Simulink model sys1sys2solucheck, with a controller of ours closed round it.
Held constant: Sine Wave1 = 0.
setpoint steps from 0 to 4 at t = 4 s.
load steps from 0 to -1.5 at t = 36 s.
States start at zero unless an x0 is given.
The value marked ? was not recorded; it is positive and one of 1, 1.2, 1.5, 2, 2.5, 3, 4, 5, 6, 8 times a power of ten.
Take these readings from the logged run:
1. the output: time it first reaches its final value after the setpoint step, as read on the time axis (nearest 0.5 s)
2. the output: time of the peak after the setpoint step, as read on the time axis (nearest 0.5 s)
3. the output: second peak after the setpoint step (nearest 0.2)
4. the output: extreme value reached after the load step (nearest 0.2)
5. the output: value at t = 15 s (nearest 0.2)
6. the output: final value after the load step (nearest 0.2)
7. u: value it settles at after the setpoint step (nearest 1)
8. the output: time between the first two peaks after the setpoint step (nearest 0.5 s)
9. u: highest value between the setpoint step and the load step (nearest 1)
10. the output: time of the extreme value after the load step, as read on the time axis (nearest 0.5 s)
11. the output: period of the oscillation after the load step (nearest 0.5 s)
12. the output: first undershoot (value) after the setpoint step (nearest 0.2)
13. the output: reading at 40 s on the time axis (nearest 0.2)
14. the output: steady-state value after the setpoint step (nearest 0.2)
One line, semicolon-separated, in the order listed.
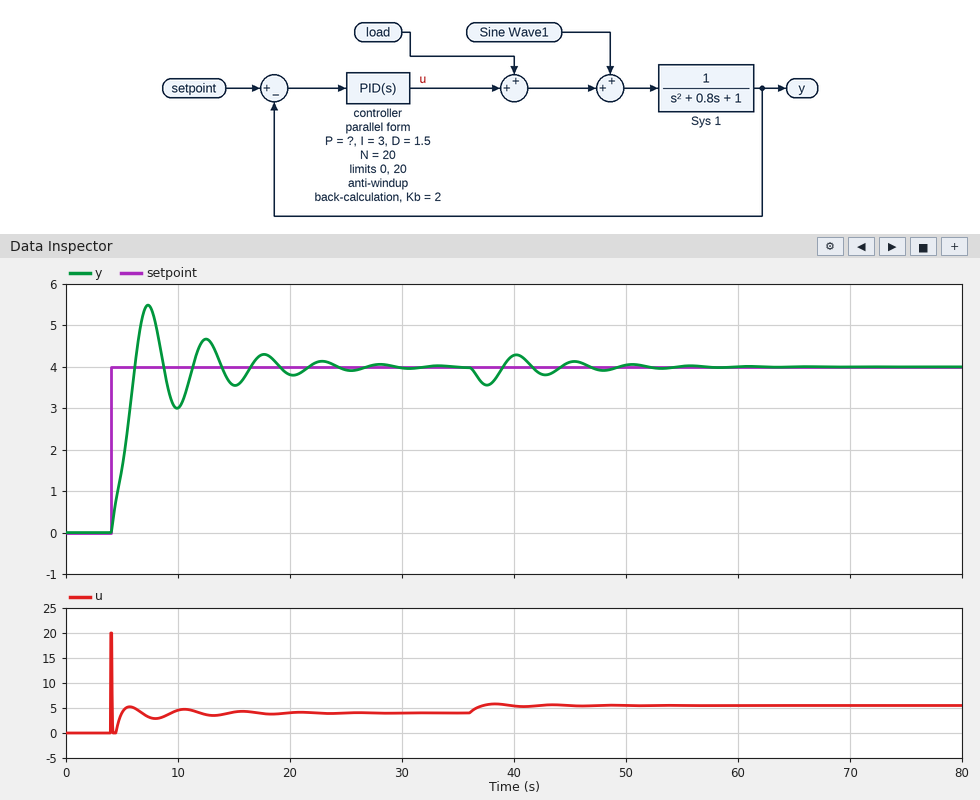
6.0 s; 7.5 s; 4.6; 3.6; 3.6; 4.0; 4; 5.0 s; 20; 37.5 s; 5.0 s; 3.0; 4.2; 4.0
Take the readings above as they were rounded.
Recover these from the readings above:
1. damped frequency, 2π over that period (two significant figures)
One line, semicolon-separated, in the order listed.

1.3 rad/s
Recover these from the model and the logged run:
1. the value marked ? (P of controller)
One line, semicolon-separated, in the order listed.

1
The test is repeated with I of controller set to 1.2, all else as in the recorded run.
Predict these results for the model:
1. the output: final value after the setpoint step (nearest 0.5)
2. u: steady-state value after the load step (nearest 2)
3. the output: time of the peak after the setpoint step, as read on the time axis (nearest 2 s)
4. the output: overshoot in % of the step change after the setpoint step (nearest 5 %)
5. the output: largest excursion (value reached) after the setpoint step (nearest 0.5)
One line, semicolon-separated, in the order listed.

4.0; 6; 10 s; 10 %; 4.5
